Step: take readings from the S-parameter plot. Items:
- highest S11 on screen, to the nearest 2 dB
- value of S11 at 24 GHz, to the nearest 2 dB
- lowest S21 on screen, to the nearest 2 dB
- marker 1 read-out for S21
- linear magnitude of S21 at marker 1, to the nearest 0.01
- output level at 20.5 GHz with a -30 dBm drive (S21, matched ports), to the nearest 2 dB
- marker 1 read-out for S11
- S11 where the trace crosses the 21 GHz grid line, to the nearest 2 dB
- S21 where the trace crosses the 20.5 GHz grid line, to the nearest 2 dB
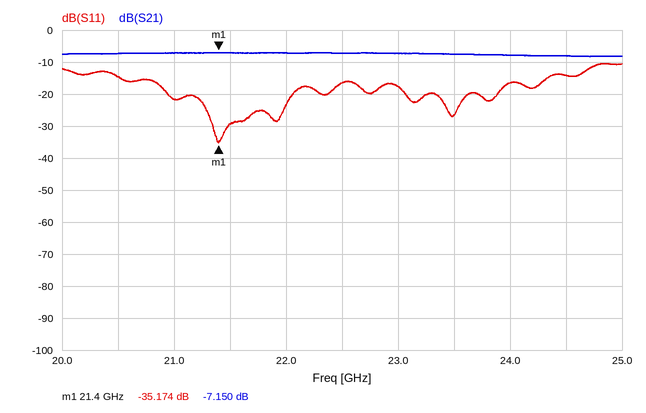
-10 dB
-16 dB
-8 dB
-7.150 dB
0.44
-38 dBm
-35.174 dB
-22 dB
-8 dB
